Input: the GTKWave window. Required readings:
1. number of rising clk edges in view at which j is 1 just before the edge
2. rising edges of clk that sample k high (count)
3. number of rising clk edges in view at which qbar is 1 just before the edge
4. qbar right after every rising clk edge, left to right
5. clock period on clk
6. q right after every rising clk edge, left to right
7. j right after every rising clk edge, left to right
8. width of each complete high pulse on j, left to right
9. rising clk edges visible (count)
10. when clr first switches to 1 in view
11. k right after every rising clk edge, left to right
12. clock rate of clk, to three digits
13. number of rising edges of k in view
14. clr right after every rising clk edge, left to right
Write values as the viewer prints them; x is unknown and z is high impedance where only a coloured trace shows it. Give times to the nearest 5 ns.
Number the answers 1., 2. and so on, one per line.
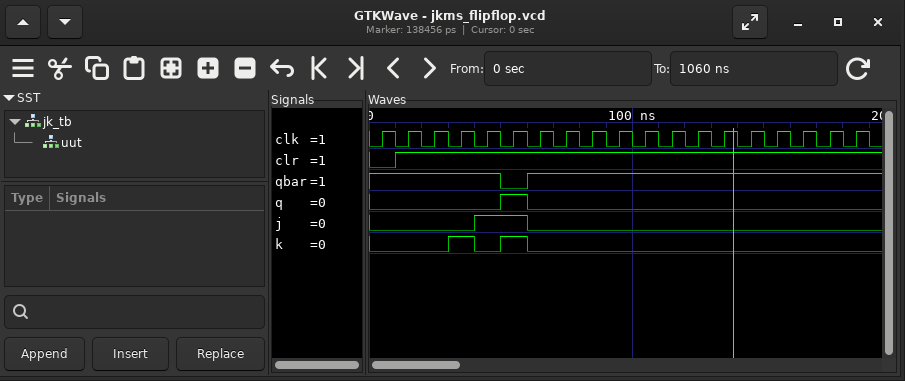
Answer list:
1. 2
2. 2
3. 18
4. 1 1 1 1 1 0 1 1 1 1 1 1 1 1 1 1 1 1 1
5. 10 ns
6. 0 0 0 0 0 1 0 0 0 0 0 0 0 0 0 0 0 0 0
7. 0 0 0 0 1 1 0 0 0 0 0 0 0 0 0 0 0 0 0
8. 20 ns
9. 19
10. 10 ns
11. 0 0 0 1 0 1 0 0 0 0 0 0 0 0 0 0 0 0 0
12. 100 MHz
13. 2
14. 0 1 1 1 1 1 1 1 1 1 1 1 1 1 1 1 1 1 1
